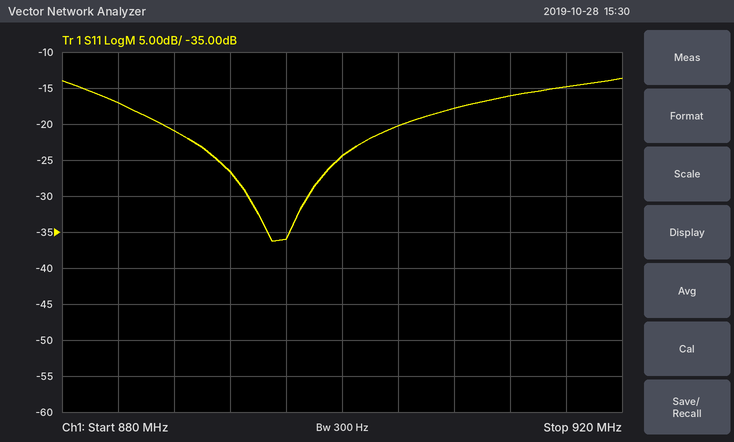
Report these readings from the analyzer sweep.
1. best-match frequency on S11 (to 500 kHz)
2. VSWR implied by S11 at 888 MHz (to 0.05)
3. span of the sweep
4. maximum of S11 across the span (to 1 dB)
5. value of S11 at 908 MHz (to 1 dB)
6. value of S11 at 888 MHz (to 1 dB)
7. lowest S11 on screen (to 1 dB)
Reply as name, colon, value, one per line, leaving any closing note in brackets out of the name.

best-match frequency on S11: 895.0 MHz
VSWR implied by S11 at 888 MHz: 1.20
span of the sweep: 40 MHz
maximum of S11 across the span: -14 dB
value of S11 at 908 MHz: -18 dB
value of S11 at 888 MHz: -21 dB
lowest S11 on screen: -36 dB
